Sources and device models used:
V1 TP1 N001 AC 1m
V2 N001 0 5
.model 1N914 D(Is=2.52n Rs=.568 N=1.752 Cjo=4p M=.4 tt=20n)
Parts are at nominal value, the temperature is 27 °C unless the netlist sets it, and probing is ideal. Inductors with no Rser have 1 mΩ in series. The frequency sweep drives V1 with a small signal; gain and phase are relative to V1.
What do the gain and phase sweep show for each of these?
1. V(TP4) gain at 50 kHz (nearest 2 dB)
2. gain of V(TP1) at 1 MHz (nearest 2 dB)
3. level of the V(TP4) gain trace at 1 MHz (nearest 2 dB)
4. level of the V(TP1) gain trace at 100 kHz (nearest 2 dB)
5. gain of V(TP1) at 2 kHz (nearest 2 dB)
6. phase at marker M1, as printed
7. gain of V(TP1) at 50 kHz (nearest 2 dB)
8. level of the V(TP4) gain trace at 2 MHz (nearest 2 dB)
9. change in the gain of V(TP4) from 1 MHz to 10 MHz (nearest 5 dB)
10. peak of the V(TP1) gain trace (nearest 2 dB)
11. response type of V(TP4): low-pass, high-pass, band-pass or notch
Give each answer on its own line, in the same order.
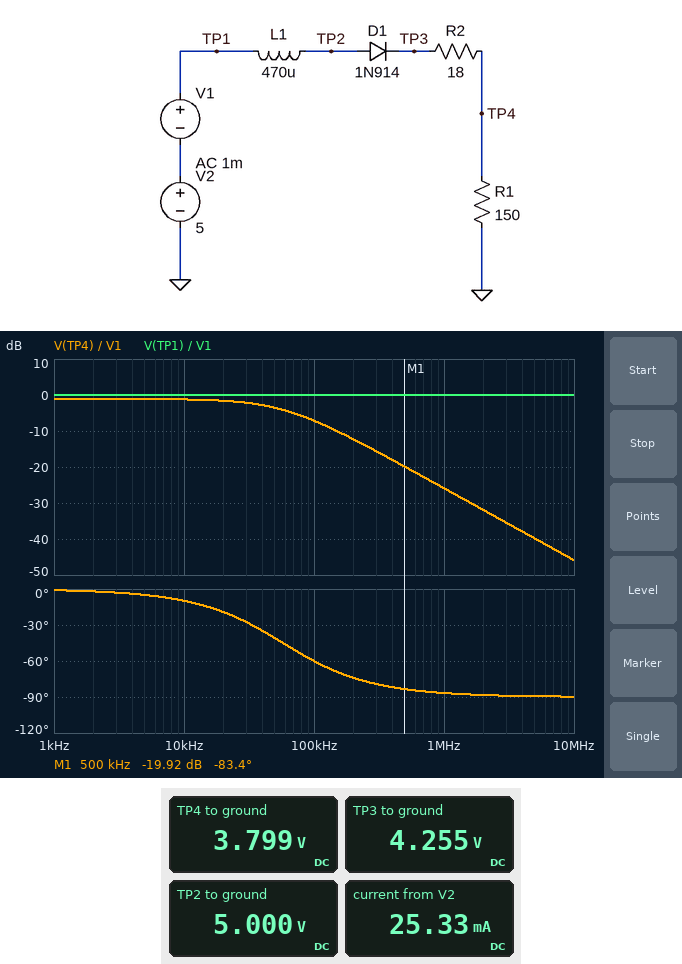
-4 dB
0 dB
-26 dB
0 dB
0 dB
-83.4 deg
0 dB
-32 dB
-20 dB
0 dB
low-pass
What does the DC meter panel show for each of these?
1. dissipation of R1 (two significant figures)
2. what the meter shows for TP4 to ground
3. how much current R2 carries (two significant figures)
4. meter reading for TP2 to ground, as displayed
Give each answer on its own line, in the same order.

96 mW
3.799 V
25 mA
5.000 V
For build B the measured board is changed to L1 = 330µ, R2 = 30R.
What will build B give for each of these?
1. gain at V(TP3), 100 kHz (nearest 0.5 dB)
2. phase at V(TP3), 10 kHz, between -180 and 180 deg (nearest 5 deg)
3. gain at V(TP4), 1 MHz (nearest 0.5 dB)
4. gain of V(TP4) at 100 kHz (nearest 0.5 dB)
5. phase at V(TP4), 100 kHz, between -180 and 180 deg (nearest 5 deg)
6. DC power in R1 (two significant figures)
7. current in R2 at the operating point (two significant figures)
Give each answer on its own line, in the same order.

-3.5 dB
-5 deg
-23.0 dB
-5.5 dB
-50 deg
84 mW
24 mA
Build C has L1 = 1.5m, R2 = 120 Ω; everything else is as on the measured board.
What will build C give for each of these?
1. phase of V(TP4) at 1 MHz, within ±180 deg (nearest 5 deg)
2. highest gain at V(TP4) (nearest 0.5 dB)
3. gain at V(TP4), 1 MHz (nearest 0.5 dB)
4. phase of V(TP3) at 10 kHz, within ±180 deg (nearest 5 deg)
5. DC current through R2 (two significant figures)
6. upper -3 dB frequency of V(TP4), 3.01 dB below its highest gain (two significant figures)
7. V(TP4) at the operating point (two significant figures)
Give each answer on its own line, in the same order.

-90 deg
-5.0 dB
-36.0 dB
-20 deg
16 mA
29 kHz
2.4 V
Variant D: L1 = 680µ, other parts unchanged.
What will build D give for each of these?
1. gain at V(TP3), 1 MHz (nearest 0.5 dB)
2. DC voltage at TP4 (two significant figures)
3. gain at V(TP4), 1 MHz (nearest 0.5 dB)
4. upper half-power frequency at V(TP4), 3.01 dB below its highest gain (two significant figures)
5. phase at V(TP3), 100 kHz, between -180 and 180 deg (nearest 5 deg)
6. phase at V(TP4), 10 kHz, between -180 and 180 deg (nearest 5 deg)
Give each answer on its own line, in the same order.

-28.0 dB
3.8 V
-29.0 dB
40 kHz
-70 deg
-15 deg
